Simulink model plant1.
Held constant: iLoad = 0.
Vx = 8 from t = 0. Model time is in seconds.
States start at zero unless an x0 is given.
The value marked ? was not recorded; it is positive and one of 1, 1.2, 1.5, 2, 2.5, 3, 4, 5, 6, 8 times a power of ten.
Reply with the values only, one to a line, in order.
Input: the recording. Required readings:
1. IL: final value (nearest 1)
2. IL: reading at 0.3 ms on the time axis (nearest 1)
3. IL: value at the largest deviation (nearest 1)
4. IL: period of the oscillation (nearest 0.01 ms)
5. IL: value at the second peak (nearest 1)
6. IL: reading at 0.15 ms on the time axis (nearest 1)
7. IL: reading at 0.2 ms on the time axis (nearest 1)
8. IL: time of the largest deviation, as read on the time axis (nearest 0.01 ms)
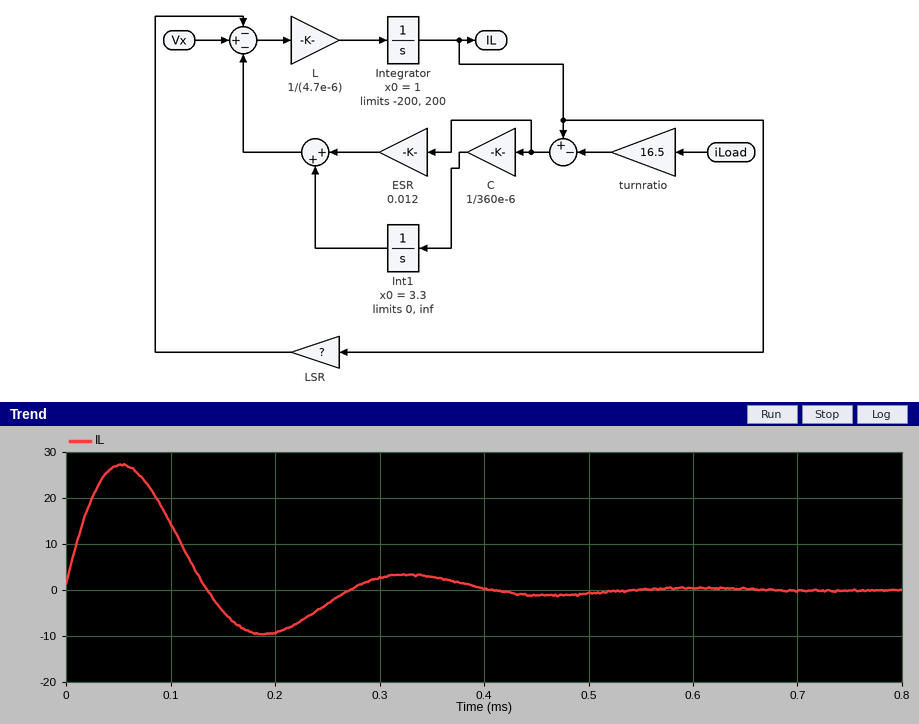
0
3
27
0.27 ms
3
-5
-9
0.05 ms
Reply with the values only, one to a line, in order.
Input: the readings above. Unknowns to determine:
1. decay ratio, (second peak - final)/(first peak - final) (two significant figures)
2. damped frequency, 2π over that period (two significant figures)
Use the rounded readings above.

0.11
23 rad/ms
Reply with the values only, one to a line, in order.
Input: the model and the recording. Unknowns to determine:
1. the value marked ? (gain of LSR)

0.06
